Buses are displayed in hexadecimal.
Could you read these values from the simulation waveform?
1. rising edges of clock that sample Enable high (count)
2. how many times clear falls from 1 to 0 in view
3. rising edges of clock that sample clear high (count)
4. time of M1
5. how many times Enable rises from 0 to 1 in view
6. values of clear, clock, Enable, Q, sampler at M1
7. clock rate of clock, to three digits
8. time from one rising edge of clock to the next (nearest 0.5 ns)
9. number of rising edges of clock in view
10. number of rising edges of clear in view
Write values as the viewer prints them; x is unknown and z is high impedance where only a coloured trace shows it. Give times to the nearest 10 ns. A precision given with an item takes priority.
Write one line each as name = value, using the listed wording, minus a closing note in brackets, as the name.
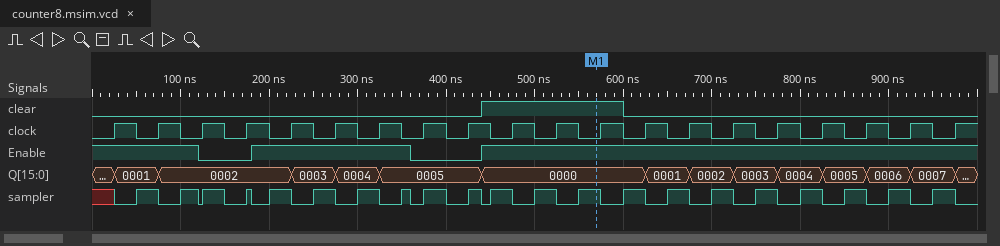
rising edges of clock that sample Enable high = 16
how many times clear falls from 1 to 0 in view = 1
rising edges of clock that sample clear high = 3
time of M1 = 570 ns
how many times Enable rises from 0 to 1 in view = 2
values of clear, clock, Enable, Q, sampler at M1 = clear=1, clock=0, Enable=1, Q=0000, sampler=1
clock rate of clock, to three digits = 20.0 MHz
time from one rising edge of clock to the next = 50 ns
number of rising edges of clock in view = 20
number of rising edges of clear in view = 1
